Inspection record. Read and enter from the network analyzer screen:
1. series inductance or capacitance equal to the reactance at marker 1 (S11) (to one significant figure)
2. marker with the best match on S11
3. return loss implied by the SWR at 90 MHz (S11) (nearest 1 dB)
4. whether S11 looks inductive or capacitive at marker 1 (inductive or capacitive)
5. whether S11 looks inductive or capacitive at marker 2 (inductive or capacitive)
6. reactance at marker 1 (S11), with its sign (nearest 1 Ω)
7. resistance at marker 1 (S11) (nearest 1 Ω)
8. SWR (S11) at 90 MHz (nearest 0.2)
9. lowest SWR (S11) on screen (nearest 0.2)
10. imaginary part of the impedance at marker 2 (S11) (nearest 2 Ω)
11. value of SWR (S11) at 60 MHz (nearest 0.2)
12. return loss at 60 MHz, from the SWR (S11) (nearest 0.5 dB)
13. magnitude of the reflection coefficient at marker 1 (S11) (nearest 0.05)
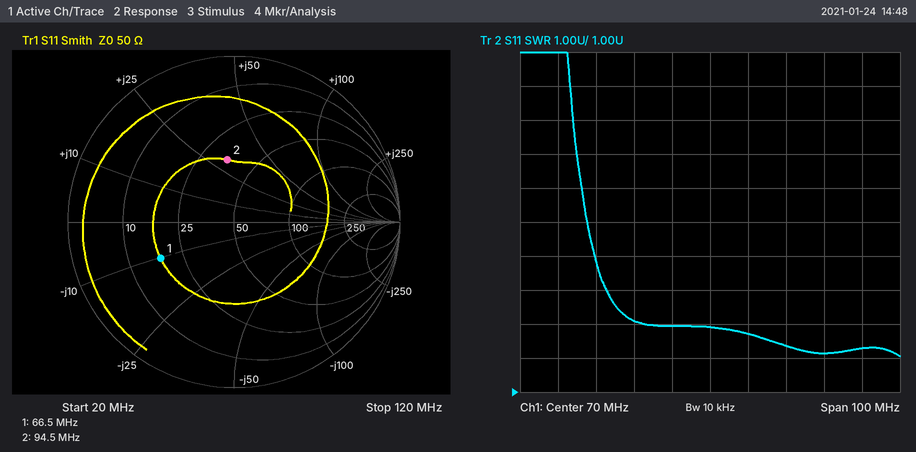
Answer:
200 pF
marker 2
8 dB
capacitive
inductive
-10 Ω
18 Ω
2.4
2.0
+30 Ω
3.0
6.0 dB
0.50
